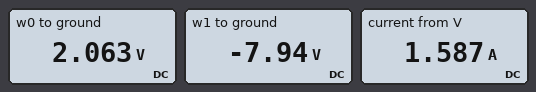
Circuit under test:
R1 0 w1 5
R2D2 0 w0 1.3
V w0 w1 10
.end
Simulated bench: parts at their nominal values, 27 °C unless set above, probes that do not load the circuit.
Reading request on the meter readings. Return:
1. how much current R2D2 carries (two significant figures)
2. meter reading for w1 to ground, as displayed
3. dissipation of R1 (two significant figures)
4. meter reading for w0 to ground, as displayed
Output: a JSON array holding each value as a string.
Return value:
["1.6 A", "-7.94 V", "13 W", "2.063 V"]
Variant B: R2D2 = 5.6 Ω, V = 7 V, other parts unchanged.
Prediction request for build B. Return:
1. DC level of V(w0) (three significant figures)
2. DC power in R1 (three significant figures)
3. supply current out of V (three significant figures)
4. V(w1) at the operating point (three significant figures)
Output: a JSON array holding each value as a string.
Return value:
["3.70 V", "2.18 W", "660 mA", "-3.30 V"]
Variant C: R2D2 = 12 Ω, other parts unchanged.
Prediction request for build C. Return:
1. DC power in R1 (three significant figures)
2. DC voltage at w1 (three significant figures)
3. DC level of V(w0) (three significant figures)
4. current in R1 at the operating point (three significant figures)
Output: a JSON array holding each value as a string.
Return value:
["1.73 W", "-2.94 V", "7.06 V", "588 mA"]
